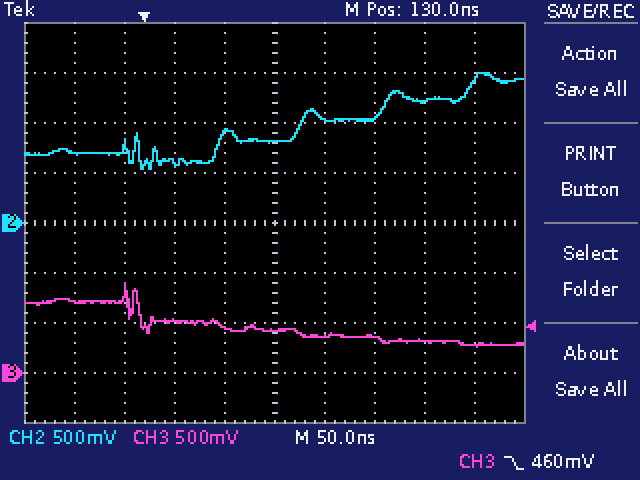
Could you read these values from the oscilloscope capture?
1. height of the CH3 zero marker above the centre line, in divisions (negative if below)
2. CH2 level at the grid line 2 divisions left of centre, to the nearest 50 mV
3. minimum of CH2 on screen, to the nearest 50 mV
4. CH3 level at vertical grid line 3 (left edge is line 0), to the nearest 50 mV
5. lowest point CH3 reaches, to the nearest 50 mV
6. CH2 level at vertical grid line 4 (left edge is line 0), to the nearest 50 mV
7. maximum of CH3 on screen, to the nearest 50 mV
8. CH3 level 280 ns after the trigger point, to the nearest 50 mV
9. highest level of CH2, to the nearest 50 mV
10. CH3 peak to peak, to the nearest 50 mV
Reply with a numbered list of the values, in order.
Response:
1. -3.0 div
2. 600 mV
3. 550 mV
4. 500 mV
5. 250 mV
6. 900 mV
7. 900 mV
8. 300 mV
9. 1.50 V
10. 650 mV
